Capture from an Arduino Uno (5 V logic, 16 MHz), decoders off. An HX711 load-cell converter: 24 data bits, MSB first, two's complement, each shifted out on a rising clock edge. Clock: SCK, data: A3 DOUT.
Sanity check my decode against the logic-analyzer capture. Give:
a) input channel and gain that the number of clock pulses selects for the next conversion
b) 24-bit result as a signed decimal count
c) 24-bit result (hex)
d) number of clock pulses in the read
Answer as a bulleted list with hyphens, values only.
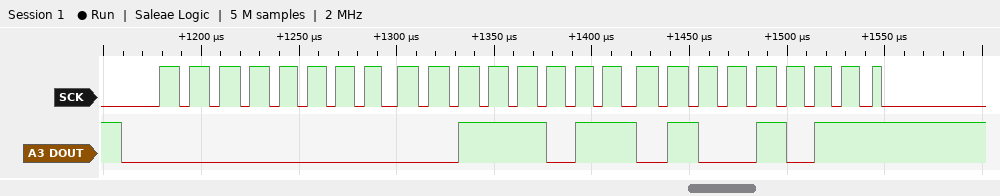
- channel A, gain 128
- 15179
- 0x003B4B
- 25
